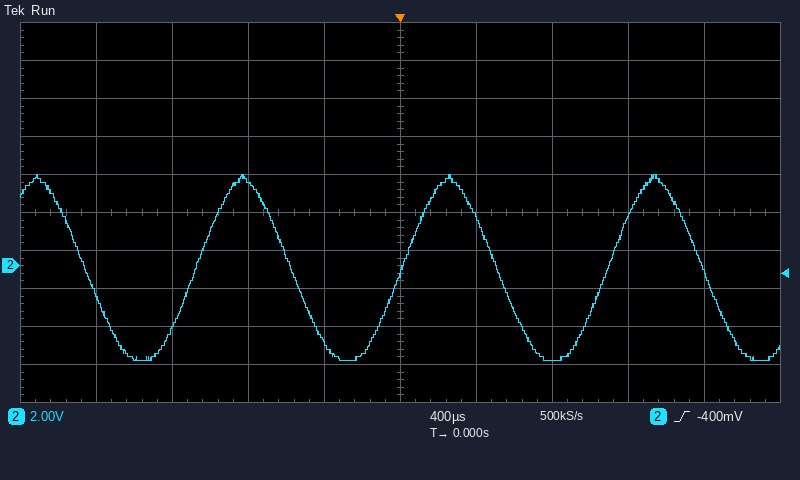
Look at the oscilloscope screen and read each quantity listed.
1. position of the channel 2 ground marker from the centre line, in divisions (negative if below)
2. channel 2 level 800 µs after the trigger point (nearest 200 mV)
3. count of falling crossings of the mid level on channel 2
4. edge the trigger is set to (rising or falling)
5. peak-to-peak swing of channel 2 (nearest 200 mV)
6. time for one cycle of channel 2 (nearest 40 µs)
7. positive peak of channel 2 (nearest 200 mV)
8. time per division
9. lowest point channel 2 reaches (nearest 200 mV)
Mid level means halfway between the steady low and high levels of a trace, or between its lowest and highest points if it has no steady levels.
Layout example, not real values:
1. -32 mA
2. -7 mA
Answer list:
1. -1.4 div
2. -5.0 V
3. 4
4. rising
5. 9.8 V
6. 1.08 ms
7. 4.8 V
8. 400 µs
9. -5.0 V
